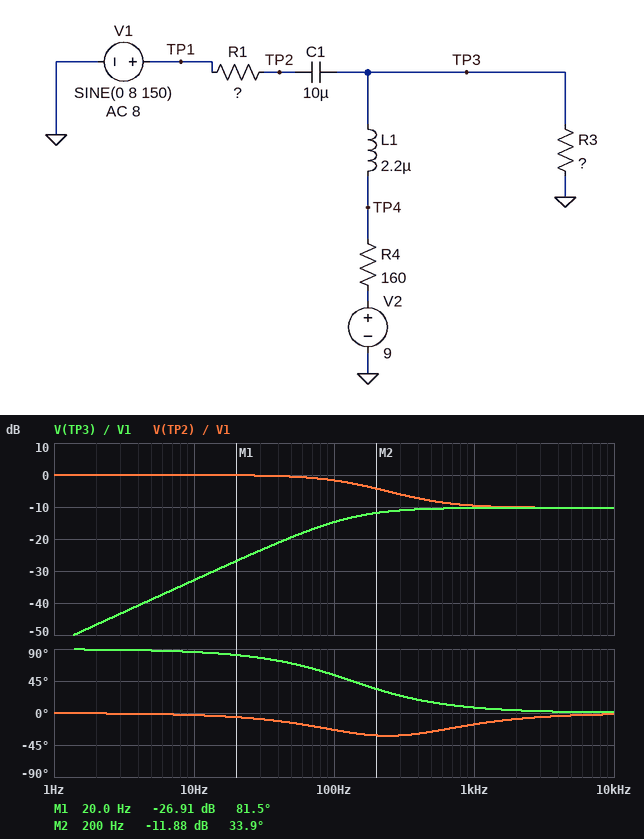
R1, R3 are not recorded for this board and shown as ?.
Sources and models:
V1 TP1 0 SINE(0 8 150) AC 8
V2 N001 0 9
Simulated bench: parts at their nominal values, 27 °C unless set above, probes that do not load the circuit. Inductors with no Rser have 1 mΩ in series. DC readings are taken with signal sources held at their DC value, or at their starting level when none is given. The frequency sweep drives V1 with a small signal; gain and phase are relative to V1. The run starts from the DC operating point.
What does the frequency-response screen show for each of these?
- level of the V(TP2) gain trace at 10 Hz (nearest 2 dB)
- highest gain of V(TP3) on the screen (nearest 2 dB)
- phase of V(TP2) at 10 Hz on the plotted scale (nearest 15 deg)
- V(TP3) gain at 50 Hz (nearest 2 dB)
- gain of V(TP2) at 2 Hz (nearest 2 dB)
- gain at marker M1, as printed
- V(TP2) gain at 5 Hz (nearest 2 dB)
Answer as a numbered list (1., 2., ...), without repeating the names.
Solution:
1. 0 dB
2. -10 dB
3. 0 deg
4. -20 dB
5. 0 dB
6. -26.91 dB
7. 0 dB
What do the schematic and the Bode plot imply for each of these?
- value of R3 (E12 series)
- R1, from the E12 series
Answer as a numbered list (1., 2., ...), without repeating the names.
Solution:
1. 47 Ω
2. 82 Ω
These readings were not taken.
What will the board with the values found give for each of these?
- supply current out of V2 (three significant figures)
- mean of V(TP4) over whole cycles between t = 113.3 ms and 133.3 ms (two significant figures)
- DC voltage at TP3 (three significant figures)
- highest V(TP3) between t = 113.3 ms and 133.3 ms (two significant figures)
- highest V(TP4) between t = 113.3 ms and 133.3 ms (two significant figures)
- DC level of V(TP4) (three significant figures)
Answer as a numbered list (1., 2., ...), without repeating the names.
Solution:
1. 43.5 mA
2. 2.0 V
3. 2.04 V
4. 3.9 V
5. 3.9 V
6. 2.04 V
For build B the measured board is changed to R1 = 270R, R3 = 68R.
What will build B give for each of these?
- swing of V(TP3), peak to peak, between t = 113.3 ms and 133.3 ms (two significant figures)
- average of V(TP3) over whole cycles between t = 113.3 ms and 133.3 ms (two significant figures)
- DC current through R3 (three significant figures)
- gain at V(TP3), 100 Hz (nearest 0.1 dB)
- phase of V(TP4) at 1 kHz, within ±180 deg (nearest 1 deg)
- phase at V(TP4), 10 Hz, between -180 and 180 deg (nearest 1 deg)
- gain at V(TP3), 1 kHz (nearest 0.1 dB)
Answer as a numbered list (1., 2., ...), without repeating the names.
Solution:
1. 2.3 V
2. 2.7 V
3. 39.5 mA
4. -17.4 dB
5. 3 deg
6. 79 deg
7. -16.5 dB
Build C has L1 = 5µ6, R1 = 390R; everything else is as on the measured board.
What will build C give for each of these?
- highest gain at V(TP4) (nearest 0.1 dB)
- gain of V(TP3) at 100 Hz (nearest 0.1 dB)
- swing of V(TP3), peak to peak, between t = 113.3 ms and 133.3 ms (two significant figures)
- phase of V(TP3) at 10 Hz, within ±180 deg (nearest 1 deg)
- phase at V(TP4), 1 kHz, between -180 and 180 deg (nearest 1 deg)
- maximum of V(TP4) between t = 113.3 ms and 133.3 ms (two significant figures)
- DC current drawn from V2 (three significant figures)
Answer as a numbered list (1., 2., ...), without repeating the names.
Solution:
1. -21.4 dB
2. -22.0 dB
3. 1.3 V
4. 75 deg
5. 2 deg
6. 2.7 V
7. 43.5 mA
